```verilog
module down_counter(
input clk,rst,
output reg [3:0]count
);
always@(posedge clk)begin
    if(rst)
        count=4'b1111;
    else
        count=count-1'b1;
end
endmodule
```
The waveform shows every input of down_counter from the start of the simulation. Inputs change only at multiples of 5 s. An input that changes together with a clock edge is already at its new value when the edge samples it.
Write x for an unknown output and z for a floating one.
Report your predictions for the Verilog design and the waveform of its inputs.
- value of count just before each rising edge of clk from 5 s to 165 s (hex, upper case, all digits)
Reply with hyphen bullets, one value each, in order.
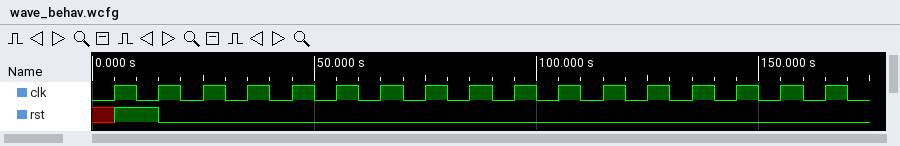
- x, F, E, D, C, B, A, 9, 8, 7, 6, 5, 4, 3, 2, 1, 0
